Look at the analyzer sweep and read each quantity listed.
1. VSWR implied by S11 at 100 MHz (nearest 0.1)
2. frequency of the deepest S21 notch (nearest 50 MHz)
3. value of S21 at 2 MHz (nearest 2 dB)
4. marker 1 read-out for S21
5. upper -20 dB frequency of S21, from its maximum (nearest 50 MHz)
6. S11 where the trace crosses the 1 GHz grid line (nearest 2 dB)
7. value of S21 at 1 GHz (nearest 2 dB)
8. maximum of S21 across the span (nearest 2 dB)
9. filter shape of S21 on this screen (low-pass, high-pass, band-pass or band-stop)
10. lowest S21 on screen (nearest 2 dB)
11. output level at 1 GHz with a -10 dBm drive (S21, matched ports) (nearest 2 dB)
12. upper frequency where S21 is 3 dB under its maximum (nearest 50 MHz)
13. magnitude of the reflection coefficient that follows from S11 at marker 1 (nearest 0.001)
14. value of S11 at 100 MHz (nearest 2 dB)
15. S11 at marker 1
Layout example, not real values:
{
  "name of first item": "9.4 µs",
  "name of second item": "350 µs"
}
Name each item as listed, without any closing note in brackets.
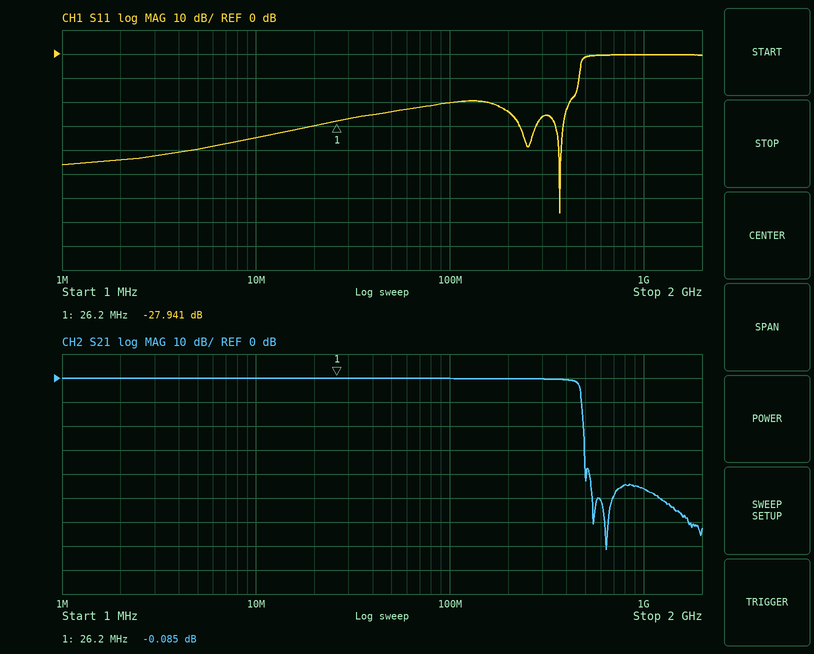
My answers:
{
  "VSWR implied by S11 at 100 MHz": "1.2",
  "frequency of the deepest S21 notch": "650 MHz",
  "value of S21 at 2 MHz": "0 dB",
  "marker 1 read-out for S21": "-0.085 dB",
  "upper -20 dB frequency of S21, from its maximum": "500 MHz",
  "S11 where the trace crosses the 1 GHz grid line": "0 dB",
  "value of S21 at 1 GHz": "-46 dB",
  "maximum of S21 across the span": "0 dB",
  "filter shape of S21 on this screen": "low-pass",
  "lowest S21 on screen": "-72 dB",
  "output level at 1 GHz with a -10 dBm drive (S21, matched ports)": "-56 dBm",
  "upper frequency where S21 is 3 dB under its maximum": "450 MHz",
  "magnitude of the reflection coefficient that follows from S11 at marker 1": "0.040",
  "value of S11 at 100 MHz": "-20 dB",
  "S11 at marker 1": "-27.941 dB"
}
